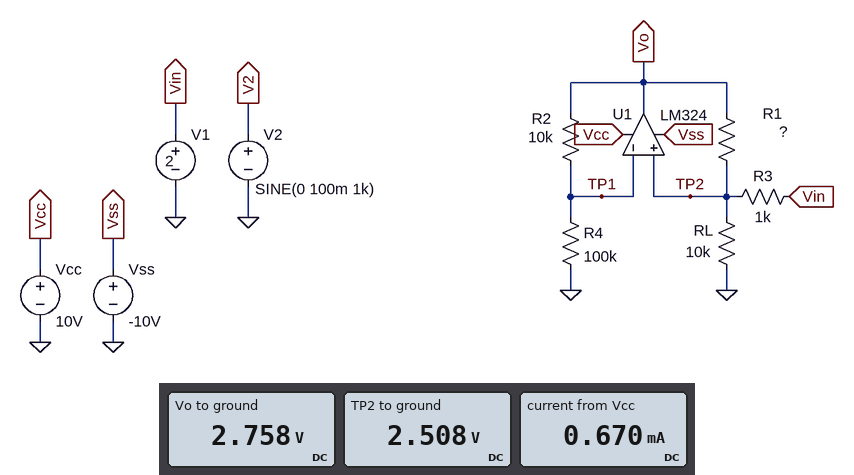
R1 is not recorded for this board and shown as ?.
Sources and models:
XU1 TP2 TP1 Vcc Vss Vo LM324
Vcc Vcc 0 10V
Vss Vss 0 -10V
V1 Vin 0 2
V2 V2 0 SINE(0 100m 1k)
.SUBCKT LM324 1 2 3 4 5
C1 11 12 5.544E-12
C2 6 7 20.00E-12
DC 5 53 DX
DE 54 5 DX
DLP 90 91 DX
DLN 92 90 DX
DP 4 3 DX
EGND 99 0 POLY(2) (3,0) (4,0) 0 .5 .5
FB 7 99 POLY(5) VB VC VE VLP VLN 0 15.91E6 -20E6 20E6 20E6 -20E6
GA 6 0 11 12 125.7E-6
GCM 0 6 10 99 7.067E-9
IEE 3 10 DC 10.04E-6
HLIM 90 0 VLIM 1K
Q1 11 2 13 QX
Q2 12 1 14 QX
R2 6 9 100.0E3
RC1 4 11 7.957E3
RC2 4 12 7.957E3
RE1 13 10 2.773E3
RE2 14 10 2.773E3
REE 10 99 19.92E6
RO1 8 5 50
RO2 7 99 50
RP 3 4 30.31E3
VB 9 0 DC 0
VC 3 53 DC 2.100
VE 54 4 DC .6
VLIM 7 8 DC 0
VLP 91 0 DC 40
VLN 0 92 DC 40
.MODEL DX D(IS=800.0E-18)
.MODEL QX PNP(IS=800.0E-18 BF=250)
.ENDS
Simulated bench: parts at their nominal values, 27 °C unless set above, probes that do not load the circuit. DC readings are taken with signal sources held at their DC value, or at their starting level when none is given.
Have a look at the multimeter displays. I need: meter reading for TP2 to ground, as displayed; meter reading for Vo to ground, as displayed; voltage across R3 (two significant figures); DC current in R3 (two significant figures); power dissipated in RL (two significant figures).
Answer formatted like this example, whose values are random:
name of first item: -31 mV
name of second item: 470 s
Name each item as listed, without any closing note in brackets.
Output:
meter reading for TP2 to ground, as displayed: 2.508 V
meter reading for Vo to ground, as displayed: 2.758 V
voltage across R3: 510 mV
DC current in R3: 510 µA
power dissipated in RL: 630 µW
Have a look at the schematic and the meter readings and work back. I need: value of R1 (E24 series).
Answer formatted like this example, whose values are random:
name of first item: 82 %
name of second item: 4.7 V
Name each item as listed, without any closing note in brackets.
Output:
value of R1: 330 Ω
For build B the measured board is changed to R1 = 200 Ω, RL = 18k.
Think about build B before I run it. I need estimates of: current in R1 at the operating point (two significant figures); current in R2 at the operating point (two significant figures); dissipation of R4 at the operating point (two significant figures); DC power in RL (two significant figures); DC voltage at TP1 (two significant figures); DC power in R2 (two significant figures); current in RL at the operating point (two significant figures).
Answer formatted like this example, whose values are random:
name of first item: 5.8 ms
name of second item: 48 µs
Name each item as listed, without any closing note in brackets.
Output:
current in R1 at the operating point: 1.8 mA
current in R2 at the operating point: 36 µA
dissipation of R4 at the operating point: 130 µW
DC power in RL: 720 µW
DC voltage at TP1: 3.6 V
DC power in R2: 13 µW
current in RL at the operating point: 200 µA
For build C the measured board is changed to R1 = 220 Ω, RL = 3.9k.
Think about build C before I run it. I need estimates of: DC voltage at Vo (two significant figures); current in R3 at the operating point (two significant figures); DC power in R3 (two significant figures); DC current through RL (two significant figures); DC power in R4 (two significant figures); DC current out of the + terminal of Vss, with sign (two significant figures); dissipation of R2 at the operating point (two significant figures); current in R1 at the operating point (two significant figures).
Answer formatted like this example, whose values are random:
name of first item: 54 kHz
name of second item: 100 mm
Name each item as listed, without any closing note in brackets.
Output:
DC voltage at Vo: 2.7 V
current in R3 at the operating point: 490 µA
DC power in R3: 240 µW
DC current through RL: 640 µA
DC power in R4: 62 µW
DC current out of the + terminal of Vss, with sign: -670 µA
dissipation of R2 at the operating point: 6.2 µW
current in R1 at the operating point: 1.1 mA
